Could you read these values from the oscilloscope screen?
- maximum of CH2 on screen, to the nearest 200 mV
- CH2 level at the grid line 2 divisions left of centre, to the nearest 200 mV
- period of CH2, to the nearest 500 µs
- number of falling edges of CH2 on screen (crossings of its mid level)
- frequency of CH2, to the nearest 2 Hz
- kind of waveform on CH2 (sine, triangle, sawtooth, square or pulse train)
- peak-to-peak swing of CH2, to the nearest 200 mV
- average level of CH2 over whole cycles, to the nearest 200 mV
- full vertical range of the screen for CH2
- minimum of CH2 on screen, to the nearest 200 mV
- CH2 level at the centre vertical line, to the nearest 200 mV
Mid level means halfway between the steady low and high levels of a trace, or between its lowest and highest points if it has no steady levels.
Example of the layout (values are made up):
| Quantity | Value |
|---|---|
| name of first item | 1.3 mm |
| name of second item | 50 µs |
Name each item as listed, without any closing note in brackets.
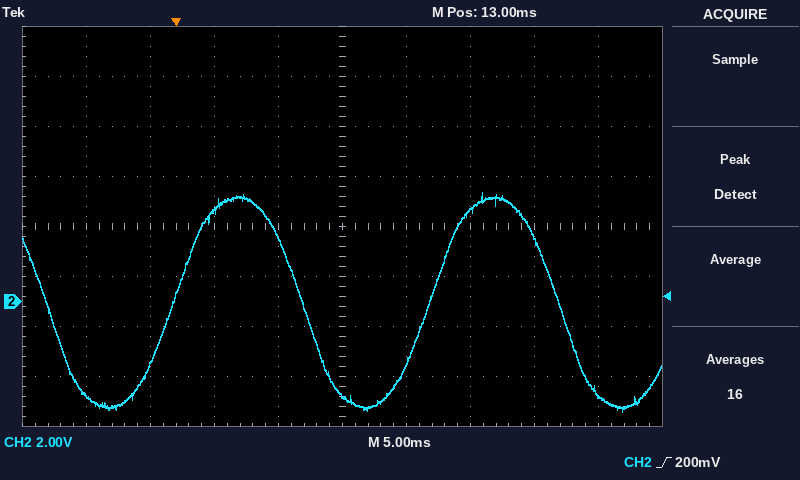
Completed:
| Quantity | Value |
|---|---|
| maximum of CH2 on screen, to the nearest 200 mV | 4.4 V |
| CH2 level at the grid line 2 divisions left of centre, to the nearest 200 mV | 3.6 V |
| period of CH2, to the nearest 500 µs | 20.0 ms |
| number of falling edges of CH2 on screen | 3 |
| frequency of CH2, to the nearest 2 Hz | 50 Hz |
| kind of waveform on CH2 | sine |
| peak-to-peak swing of CH2, to the nearest 200 mV | 8.8 V |
| average level of CH2 over whole cycles, to the nearest 200 mV | 0.0 V |
| full vertical range of the screen for CH2 | 16 V |
| minimum of CH2 on screen, to the nearest 200 mV | -4.4 V |
| CH2 level at the centre vertical line, to the nearest 200 mV | -3.8 V |
